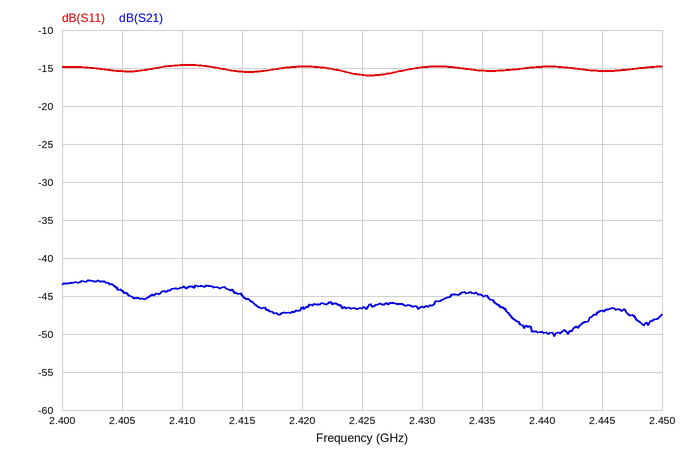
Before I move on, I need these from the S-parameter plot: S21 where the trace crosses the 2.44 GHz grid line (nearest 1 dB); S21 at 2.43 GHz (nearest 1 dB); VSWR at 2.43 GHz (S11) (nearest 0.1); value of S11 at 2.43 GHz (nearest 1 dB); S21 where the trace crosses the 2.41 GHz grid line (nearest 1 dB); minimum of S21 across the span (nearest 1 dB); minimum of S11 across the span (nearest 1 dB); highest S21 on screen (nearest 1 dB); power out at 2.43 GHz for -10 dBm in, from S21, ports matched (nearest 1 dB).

-50 dB
-46 dB
1.4
-15 dB
-44 dB
-50 dB
-16 dB
-43 dB
-56 dBm
